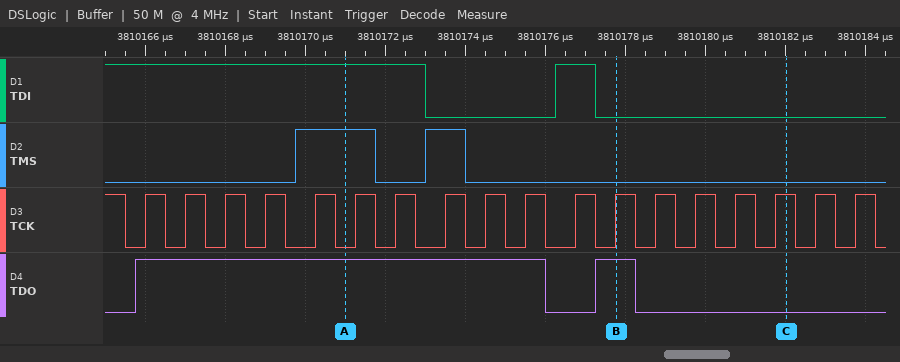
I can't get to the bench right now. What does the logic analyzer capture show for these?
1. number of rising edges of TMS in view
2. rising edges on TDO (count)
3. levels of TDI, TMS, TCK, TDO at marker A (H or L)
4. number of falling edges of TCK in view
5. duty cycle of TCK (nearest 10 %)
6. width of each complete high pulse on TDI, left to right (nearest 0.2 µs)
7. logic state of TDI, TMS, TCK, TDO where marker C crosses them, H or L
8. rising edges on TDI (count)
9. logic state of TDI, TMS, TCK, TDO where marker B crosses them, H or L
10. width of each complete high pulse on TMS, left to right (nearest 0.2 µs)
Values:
2
2
TDI=H, TMS=H, TCK=L, TDO=H
19
50 %
1 µs
TDI=L, TMS=L, TCK=H, TDO=L
1
TDI=L, TMS=L, TCK=H, TDO=H
2 µs, 1 µs
